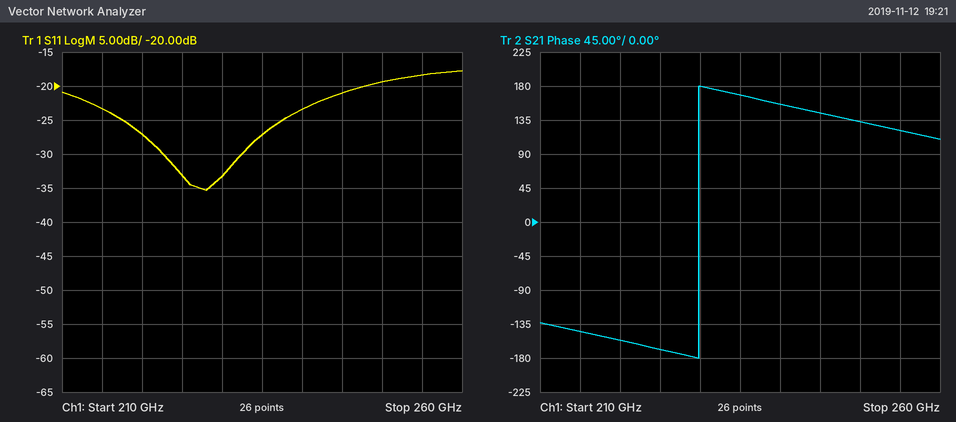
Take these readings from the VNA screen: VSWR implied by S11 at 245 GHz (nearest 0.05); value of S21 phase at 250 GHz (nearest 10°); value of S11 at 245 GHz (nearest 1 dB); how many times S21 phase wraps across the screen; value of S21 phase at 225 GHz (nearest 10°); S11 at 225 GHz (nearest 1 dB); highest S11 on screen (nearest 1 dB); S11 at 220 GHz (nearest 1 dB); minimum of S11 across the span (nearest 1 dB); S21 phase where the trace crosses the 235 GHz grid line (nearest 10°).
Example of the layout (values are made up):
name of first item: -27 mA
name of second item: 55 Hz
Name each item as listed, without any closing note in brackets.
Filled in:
VSWR implied by S11 at 245 GHz: 1.20
value of S21 phase at 250 GHz: 130°
value of S11 at 245 GHz: -21 dB
how many times S21 phase wraps across the screen: 1
value of S21 phase at 225 GHz: -170°
S11 at 225 GHz: -33 dB
highest S11 on screen: -18 dB
S11 at 220 GHz: -27 dB
minimum of S11 across the span: -35 dB
S21 phase where the trace crosses the 235 GHz grid line: 170°
